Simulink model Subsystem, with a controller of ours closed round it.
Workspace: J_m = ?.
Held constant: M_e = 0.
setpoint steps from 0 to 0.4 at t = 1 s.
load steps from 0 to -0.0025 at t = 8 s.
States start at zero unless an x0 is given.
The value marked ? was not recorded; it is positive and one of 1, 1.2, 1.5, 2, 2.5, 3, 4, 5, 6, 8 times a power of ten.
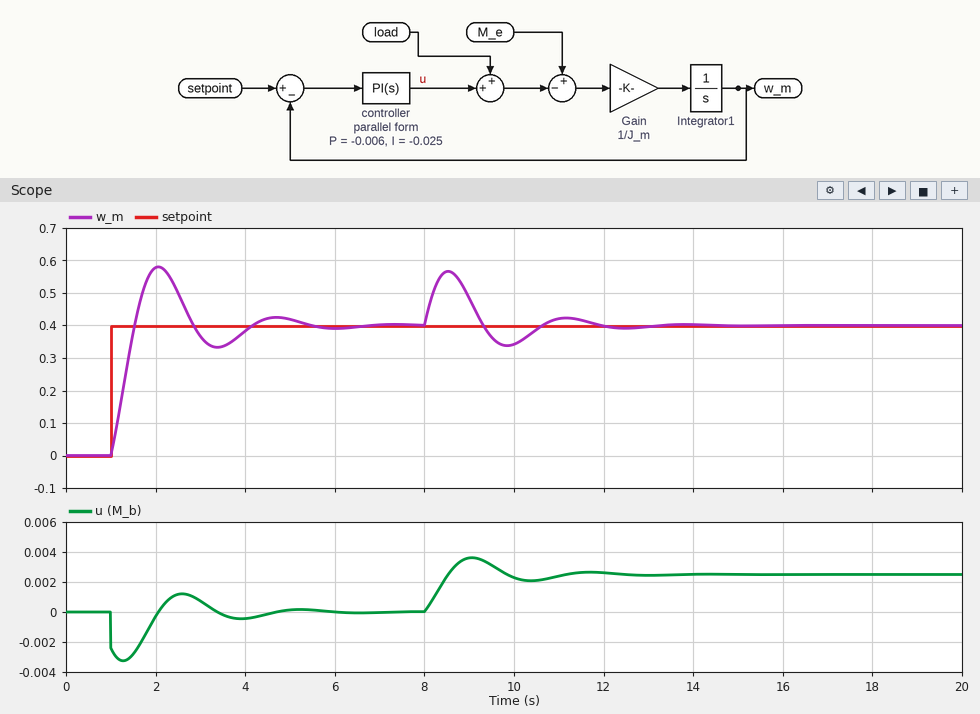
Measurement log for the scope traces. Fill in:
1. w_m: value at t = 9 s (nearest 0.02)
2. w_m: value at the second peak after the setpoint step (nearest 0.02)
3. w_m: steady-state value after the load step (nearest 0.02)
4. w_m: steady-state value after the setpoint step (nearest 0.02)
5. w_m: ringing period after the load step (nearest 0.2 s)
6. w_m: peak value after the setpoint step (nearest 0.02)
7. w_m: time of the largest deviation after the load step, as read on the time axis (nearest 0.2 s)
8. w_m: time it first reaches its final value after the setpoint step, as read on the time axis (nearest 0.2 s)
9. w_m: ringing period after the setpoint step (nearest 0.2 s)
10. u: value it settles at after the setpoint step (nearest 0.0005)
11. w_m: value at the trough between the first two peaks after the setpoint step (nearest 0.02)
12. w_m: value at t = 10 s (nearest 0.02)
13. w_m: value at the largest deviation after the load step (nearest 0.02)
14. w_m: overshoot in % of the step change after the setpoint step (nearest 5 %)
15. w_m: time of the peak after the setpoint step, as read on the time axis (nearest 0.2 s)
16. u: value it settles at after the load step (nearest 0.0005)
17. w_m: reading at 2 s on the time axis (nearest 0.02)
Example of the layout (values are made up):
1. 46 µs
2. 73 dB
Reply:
1. 0.48
2. 0.42
3. 0.40
4. 0.40
5. 2.6 s
6. 0.58
7. 8.6 s
8. 1.6 s
9. 2.6 s
10. 0.0000
11. 0.34
12. 0.34
13. 0.56
14. 45 %
15. 2.0 s
16. 0.0025
17. 0.58
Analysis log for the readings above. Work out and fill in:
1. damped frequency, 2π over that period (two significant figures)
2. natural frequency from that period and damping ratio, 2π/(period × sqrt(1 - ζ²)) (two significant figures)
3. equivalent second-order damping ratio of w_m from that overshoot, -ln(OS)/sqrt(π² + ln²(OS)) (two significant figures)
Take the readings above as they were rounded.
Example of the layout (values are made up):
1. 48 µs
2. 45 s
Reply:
1. 2.4 rad/s
2. 2.5 rad/s
3. 0.25
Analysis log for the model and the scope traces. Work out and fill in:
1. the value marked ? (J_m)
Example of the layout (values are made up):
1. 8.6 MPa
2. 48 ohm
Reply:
1. 0.004
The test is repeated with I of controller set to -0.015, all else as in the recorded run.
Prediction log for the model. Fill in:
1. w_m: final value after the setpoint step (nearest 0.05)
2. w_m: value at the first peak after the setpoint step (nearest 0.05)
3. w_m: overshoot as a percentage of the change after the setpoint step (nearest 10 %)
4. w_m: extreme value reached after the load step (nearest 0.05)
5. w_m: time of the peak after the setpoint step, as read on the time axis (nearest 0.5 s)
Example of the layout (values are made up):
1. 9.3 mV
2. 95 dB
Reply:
1. 0.40
2. 0.55
3. 40 %
4. 0.60
5. 2.5 s
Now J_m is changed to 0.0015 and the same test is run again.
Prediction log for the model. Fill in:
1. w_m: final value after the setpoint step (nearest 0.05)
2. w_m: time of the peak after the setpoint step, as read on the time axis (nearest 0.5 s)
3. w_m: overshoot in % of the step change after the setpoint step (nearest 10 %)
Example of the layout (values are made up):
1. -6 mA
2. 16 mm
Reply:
1. 0.40
2. 1.5 s
3. 30 %
